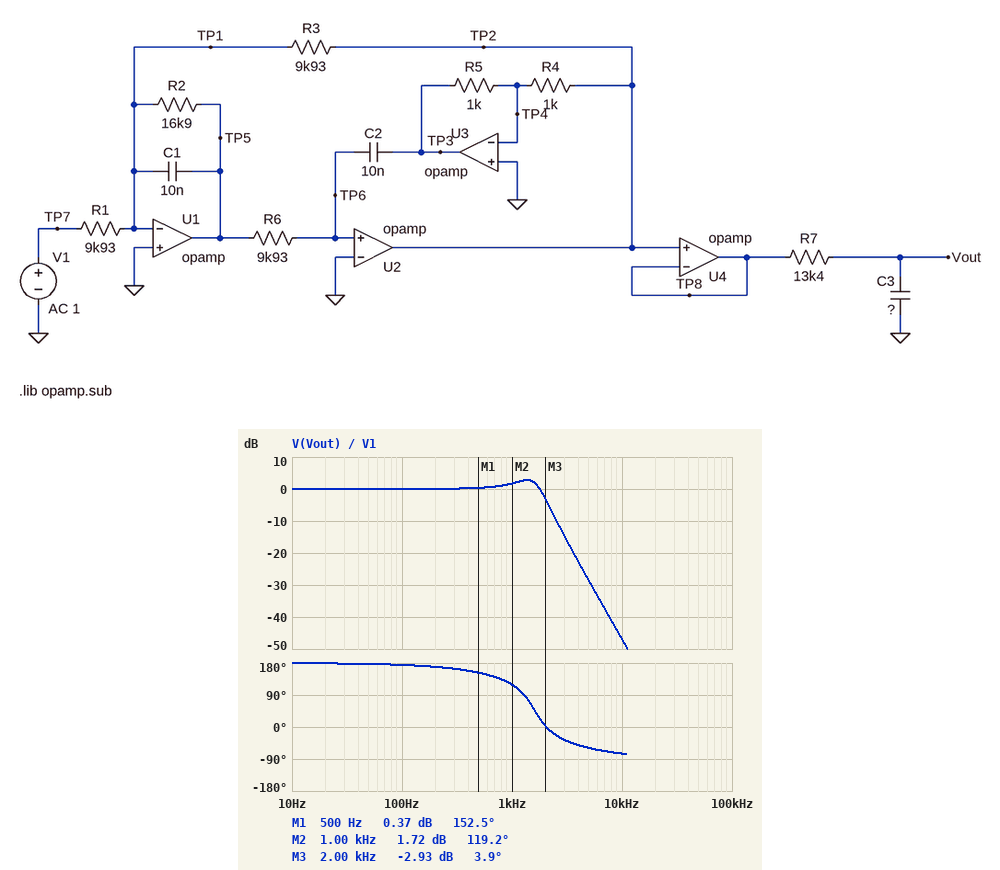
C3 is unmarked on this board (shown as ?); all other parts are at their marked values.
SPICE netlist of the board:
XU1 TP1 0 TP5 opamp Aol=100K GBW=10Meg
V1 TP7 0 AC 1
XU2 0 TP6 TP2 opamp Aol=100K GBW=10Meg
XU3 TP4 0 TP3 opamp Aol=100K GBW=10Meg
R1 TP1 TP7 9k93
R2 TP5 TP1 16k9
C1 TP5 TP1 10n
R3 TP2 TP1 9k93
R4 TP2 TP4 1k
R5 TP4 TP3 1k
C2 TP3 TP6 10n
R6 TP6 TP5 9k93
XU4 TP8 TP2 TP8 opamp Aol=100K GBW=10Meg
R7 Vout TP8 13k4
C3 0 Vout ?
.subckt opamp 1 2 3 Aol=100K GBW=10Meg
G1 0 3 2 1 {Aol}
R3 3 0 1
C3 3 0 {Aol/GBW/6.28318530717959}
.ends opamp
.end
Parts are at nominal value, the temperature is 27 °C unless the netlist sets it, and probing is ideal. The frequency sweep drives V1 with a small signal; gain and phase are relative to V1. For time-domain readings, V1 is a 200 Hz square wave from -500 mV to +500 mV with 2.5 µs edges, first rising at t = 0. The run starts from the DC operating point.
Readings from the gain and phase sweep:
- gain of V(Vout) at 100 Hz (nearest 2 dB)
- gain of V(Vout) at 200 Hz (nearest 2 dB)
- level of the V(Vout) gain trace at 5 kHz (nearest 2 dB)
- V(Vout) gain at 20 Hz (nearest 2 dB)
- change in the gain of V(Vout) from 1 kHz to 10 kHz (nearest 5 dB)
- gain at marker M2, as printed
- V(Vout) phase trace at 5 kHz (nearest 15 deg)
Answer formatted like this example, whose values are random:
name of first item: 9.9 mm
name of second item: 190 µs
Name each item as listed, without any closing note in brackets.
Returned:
gain of V(Vout) at 100 Hz: 0 dB
gain of V(Vout) at 200 Hz: 0 dB
level of the V(Vout) gain trace at 5 kHz: -28 dB
V(Vout) gain at 20 Hz: 0 dB
change in the gain of V(Vout) from 1 kHz to 10 kHz: -50 dB
gain at marker M2, as printed: 1.72 dB
V(Vout) phase trace at 5 kHz: -60 deg
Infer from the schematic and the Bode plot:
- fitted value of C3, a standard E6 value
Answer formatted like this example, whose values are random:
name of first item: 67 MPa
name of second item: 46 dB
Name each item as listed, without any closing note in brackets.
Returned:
fitted value of C3, a standard E6 value: 6.8 nF
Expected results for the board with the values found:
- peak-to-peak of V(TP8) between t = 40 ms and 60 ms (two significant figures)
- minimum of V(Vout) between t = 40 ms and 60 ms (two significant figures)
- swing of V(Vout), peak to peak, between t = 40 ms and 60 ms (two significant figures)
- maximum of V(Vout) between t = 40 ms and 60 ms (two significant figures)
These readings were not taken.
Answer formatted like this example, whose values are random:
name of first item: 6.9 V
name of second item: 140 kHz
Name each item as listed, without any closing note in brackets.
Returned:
peak-to-peak of V(TP8) between t = 40 ms and 60 ms: 1.8 V
minimum of V(Vout) between t = 40 ms and 60 ms: -750 mV
swing of V(Vout), peak to peak, between t = 40 ms and 60 ms: 1.5 V
maximum of V(Vout) between t = 40 ms and 60 ms: 750 mV
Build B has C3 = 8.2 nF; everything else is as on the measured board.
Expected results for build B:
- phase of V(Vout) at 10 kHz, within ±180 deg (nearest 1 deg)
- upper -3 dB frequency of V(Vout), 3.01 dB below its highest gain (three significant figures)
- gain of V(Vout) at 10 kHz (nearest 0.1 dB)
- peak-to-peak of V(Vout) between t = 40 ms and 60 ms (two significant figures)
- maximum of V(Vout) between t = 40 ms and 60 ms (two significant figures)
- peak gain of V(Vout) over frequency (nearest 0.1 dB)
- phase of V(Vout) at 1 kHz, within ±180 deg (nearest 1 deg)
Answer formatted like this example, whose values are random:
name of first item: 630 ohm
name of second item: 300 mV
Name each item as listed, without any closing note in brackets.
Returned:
phase of V(Vout) at 10 kHz, within ±180 deg: -76 deg
upper -3 dB frequency of V(Vout), 3.01 dB below its highest gain: 1.79 kHz
gain of V(Vout) at 10 kHz: -48.5 dB
peak-to-peak of V(Vout) between t = 40 ms and 60 ms: 1.4 V
maximum of V(Vout) between t = 40 ms and 60 ms: 710 mV
peak gain of V(Vout) over frequency: 2.1 dB
phase of V(Vout) at 1 kHz, within ±180 deg: 114 deg
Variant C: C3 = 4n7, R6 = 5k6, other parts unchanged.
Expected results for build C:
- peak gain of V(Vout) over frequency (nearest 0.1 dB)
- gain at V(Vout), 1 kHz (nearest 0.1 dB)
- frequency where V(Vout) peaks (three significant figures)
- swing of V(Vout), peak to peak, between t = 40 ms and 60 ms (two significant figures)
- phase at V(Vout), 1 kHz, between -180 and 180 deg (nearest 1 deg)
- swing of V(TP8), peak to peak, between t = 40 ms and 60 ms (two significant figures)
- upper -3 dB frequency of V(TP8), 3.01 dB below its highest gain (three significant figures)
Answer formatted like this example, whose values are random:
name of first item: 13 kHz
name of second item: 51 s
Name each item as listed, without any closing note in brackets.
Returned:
peak gain of V(Vout) over frequency: 5.2 dB
gain at V(Vout), 1 kHz: 1.2 dB
frequency where V(Vout) peaks: 1.98 kHz
swing of V(Vout), peak to peak, between t = 40 ms and 60 ms: 1.7 V
phase at V(Vout), 1 kHz, between -180 and 180 deg: 144 deg
swing of V(TP8), peak to peak, between t = 40 ms and 60 ms: 2.0 V
upper -3 dB frequency of V(TP8), 3.01 dB below its highest gain: 2.46 kHz
